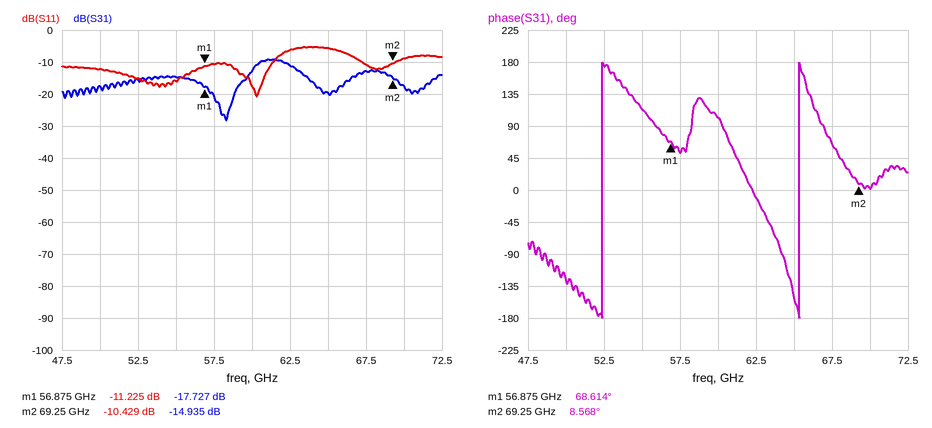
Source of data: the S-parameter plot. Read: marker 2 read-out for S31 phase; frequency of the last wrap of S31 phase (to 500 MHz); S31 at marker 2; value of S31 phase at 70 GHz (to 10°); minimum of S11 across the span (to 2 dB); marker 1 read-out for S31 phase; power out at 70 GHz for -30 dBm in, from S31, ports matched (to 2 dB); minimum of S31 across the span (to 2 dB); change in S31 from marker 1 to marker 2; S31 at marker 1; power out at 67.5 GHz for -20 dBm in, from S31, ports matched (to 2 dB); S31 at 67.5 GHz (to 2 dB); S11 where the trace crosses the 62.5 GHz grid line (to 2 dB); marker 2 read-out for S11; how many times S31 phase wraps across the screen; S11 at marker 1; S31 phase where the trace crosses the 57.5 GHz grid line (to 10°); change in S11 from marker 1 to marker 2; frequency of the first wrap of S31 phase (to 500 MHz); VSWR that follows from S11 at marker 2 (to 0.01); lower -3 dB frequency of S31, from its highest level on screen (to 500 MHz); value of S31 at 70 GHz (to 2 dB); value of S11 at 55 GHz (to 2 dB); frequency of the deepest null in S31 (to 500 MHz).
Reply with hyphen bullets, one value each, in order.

- 8.568°
- 65.5 GHz
- -14.935 dB
- 0°
- -20 dB
- 68.614°
- -48 dBm
- -28 dB
- 2.792 dB
- -17.727 dB
- -32 dBm
- -12 dB
- -6 dB
- -10.429 dB
- 2
- -11.225 dB
- 50°
- 0.796 dB
- 52.5 GHz
- 1.86
- 60.0 GHz
- -18 dB
- -16 dB
- 58.5 GHz
